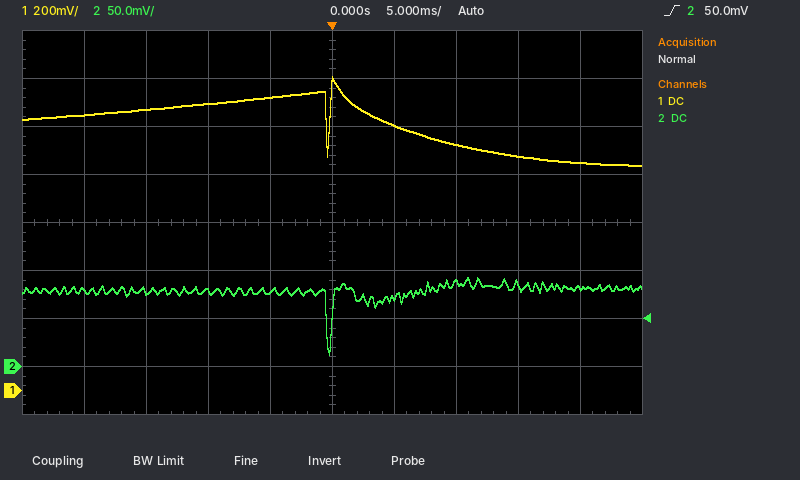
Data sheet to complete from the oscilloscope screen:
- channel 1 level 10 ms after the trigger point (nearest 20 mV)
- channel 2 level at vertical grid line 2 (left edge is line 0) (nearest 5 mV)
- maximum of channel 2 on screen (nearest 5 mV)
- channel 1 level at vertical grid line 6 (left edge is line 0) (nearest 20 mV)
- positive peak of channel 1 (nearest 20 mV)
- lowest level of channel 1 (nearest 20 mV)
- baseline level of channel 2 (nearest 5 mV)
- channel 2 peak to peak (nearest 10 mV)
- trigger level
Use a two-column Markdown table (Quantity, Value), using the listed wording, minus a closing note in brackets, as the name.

| Quantity | Value |
|---|---|
| channel 1 level 10 ms after the trigger point | 1.02 V |
| channel 2 level at vertical grid line 2 (left edge is line 0) | 80 mV |
| maximum of channel 2 on screen | 95 mV |
| channel 1 level at vertical grid line 6 (left edge is line 0) | 1.10 V |
| positive peak of channel 1 | 1.30 V |
| lowest level of channel 1 | 940 mV |
| baseline level of channel 2 | 80 mV |
| channel 2 peak to peak | 80 mV |
| trigger level | 50.0 mV |
